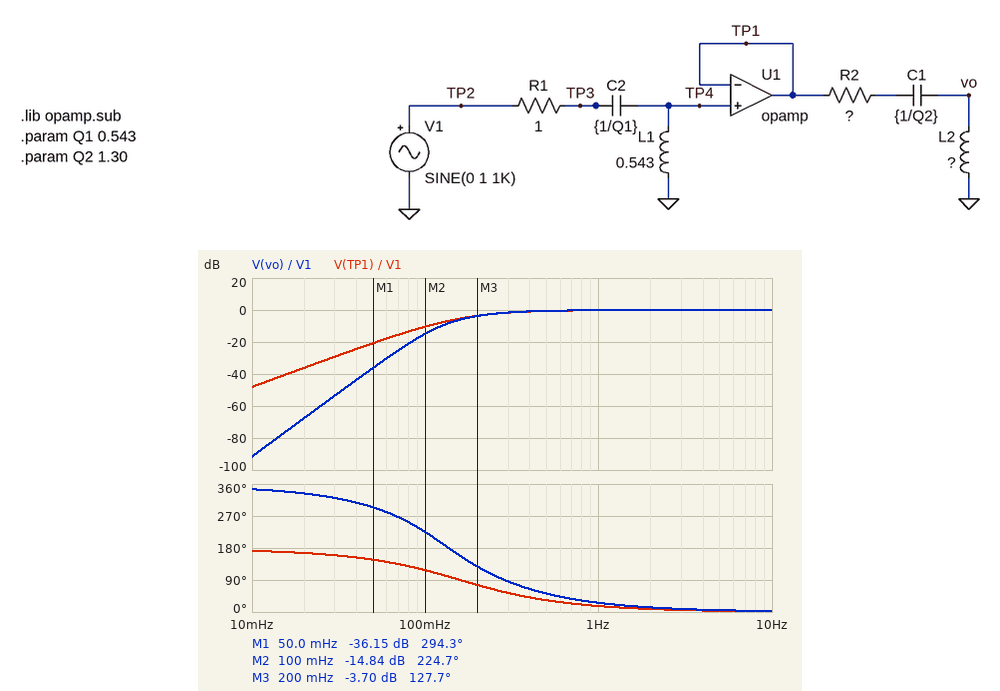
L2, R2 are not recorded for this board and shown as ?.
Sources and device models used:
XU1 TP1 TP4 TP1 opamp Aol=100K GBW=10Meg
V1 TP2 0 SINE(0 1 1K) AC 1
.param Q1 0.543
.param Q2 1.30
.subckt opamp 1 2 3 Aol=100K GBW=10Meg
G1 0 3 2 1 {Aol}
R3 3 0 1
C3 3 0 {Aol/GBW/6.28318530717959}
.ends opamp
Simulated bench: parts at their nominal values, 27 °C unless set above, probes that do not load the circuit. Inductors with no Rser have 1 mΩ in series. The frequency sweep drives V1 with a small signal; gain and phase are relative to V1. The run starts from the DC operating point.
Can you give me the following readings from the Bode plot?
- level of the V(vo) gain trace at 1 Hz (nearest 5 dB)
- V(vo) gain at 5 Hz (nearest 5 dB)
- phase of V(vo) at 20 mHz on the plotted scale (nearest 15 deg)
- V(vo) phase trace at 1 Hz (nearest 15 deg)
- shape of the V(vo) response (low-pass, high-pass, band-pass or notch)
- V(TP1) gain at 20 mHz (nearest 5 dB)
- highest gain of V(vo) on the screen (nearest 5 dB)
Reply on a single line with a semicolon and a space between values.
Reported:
0 dB; 0 dB; 330 deg; 30 deg; high-pass; -35 dB; 0 dB
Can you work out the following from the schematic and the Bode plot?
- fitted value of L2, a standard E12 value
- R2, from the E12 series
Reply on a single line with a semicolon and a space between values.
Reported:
2.2 H; 2.2 Ω
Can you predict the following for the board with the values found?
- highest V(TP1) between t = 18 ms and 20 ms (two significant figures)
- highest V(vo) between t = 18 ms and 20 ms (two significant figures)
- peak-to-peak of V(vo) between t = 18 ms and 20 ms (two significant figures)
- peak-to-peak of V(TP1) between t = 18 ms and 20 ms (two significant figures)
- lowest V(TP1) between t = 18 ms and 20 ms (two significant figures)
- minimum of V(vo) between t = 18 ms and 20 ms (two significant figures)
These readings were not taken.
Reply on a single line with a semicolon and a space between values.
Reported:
1.0 V; 1.0 V; 2.0 V; 2.0 V; -1.0 V; -1.0 V
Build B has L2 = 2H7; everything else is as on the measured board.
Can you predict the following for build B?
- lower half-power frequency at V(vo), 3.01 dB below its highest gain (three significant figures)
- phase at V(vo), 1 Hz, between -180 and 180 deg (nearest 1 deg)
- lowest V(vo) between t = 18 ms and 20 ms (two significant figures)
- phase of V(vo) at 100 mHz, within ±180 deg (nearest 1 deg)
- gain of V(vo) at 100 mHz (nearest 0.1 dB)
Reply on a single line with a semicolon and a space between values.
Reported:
205 mHz; 24 deg; -1.0 V; -143 deg; -12.8 dB
